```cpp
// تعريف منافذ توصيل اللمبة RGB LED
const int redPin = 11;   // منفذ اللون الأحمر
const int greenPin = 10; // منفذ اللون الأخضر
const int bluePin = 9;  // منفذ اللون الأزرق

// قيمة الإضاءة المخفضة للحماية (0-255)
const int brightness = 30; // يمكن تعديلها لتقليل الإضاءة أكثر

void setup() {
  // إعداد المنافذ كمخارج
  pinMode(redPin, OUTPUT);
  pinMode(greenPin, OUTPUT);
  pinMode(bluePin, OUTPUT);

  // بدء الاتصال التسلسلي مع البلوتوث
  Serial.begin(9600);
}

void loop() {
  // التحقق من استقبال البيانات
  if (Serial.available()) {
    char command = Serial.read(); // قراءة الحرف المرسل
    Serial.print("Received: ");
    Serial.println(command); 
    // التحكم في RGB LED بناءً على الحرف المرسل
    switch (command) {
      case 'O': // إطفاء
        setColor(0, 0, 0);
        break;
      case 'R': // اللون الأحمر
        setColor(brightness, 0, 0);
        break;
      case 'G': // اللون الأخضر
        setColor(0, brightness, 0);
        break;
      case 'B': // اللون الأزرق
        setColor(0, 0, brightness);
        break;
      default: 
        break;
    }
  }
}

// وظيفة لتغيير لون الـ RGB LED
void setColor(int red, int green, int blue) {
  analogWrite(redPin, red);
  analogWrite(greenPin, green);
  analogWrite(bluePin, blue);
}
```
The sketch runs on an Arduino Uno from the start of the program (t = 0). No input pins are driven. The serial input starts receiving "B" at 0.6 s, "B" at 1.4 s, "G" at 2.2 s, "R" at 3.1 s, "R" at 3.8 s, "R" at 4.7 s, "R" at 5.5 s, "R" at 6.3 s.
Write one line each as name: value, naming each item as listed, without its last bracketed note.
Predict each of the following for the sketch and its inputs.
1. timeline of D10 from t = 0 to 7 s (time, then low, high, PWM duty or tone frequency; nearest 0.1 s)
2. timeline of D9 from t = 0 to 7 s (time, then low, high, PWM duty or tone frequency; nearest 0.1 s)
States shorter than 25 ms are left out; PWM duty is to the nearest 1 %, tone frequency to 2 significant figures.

timeline of D10 from t = 0 to 7 s: 0 s low; 2.2 s PWM 12 %; 3.1 s low
timeline of D9 from t = 0 to 7 s: 0 s low; 0.6 s PWM 12 %; 2.2 s low
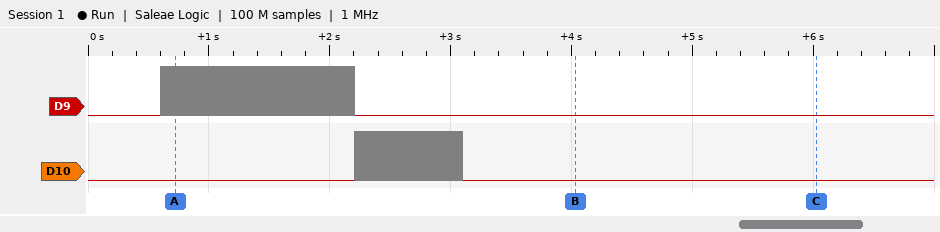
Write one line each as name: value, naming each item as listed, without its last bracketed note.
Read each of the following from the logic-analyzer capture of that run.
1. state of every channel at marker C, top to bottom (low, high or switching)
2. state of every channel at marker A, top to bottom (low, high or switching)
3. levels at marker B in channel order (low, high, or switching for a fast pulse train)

state of every channel at marker C, top to bottom: D9 low, D10 low
state of every channel at marker A, top to bottom: D9 switching, D10 low
levels at marker B in channel order: D9 low, D10 low
